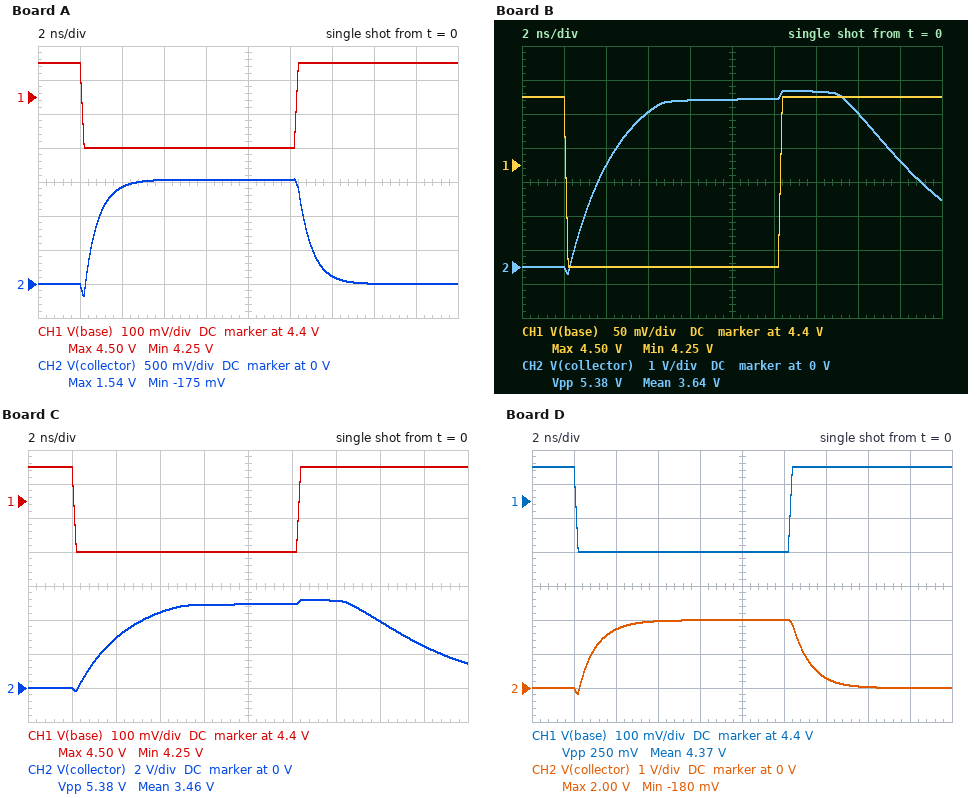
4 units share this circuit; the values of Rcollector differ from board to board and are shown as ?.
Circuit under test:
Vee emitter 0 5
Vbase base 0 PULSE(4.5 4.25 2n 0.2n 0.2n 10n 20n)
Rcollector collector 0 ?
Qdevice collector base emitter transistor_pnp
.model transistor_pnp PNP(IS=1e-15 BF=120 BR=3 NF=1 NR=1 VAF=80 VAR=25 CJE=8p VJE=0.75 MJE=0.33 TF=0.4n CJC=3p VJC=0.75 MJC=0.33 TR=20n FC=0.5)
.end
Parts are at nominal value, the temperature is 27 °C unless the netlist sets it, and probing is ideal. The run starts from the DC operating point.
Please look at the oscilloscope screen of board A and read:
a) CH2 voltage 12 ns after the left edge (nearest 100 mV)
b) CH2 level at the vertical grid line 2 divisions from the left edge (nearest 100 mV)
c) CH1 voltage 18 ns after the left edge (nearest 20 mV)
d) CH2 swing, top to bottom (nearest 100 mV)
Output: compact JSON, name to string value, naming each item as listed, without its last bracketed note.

{"CH2 voltage 12 ns after the left edge": "1.5 V", "CH2 level at the vertical grid line 2 divisions from the left edge": "1.4 V", "CH1 voltage 18 ns after the left edge": "4.50 V", "CH2 swing, top to bottom": "1.7 V"}
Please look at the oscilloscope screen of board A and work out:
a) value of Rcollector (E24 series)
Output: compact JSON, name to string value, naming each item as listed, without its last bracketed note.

{"value of Rcollector": "390 Ω"}
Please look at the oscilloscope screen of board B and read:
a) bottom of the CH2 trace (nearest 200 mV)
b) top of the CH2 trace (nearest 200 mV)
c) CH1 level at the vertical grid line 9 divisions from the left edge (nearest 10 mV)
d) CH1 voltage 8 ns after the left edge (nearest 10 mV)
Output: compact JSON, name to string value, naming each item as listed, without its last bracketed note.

{"bottom of the CH2 trace": "-200 mV", "top of the CH2 trace": "5.2 V", "CH1 level at the vertical grid line 9 divisions from the left edge": "4.50 V", "CH1 voltage 8 ns after the left edge": "4.25 V"}
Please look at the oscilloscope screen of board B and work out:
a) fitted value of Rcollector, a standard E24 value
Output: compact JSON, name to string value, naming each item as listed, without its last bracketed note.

{"fitted value of Rcollector, a standard E24 value": "2.2 kΩ"}
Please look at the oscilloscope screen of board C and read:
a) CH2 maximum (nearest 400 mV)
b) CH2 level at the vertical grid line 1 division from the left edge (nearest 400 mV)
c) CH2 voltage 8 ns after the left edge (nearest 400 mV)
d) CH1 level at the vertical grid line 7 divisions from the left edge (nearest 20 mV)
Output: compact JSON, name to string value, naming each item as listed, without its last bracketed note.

{"CH2 maximum": "5.2 V", "CH2 level at the vertical grid line 1 division from the left edge": "0 V", "CH2 voltage 8 ns after the left edge": "4.8 V", "CH1 level at the vertical grid line 7 divisions from the left edge": "4.50 V"}
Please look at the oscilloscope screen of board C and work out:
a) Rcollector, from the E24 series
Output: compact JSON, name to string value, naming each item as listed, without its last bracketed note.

{"Rcollector, from the E24 series": "2 kΩ"}
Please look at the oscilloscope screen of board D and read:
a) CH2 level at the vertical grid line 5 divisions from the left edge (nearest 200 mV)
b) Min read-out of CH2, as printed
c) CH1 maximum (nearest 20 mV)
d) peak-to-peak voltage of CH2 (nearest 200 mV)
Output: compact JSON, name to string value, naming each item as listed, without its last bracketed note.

{"CH2 level at the vertical grid line 5 divisions from the left edge": "2.0 V", "Min read-out of CH2, as printed": "-180 mV", "CH1 maximum": "4.50 V", "peak-to-peak voltage of CH2": "2.2 V"}
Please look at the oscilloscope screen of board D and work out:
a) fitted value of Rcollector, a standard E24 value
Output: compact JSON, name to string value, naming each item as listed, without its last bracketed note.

{"fitted value of Rcollector, a standard E24 value": "510 Ω"}
